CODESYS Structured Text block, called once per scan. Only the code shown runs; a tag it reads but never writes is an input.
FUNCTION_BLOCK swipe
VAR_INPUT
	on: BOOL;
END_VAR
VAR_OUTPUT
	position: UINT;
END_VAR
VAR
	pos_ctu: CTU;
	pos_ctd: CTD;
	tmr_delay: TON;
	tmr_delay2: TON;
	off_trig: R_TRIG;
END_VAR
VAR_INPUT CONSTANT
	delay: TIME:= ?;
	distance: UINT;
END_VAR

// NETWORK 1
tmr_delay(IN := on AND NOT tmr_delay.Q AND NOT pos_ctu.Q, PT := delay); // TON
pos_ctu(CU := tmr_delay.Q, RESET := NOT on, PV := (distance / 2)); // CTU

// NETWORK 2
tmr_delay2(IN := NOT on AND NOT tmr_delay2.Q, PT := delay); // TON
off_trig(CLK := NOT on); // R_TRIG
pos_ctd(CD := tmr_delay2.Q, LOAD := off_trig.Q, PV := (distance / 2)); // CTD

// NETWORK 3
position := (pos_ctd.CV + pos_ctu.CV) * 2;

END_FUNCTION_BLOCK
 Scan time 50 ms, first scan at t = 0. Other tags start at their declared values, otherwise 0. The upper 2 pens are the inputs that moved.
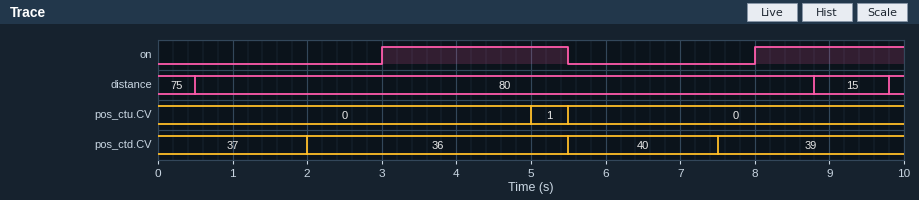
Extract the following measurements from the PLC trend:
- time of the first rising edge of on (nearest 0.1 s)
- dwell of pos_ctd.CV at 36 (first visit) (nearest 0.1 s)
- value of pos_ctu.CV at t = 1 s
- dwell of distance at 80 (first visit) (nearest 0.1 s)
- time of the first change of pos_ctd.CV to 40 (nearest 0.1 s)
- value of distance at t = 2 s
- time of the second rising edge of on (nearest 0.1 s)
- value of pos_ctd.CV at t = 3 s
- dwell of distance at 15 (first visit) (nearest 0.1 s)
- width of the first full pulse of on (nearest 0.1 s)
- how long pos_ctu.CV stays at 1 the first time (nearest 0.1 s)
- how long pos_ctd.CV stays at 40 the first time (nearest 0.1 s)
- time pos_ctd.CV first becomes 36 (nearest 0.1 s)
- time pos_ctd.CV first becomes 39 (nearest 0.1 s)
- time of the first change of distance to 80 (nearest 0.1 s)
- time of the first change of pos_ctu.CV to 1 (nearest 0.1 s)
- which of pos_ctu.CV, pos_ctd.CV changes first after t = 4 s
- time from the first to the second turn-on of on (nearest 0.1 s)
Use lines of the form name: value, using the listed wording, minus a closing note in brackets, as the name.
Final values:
time of the first rising edge of on: 3.0 s
dwell of pos_ctd.CV at 36 (first visit): 3.5 s
value of pos_ctu.CV at t = 1 s: 0
dwell of distance at 80 (first visit): 8.3 s
time of the first change of pos_ctd.CV to 40: 5.5 s
value of distance at t = 2 s: 80
time of the second rising edge of on: 8.0 s
value of pos_ctd.CV at t = 3 s: 36
dwell of distance at 15 (first visit): 1.0 s
width of the first full pulse of on: 2.5 s
how long pos_ctu.CV stays at 1 the first time: 0.5 s
how long pos_ctd.CV stays at 40 the first time: 2.0 s
time pos_ctd.CV first becomes 36: 2.0 s
time pos_ctd.CV first becomes 39: 7.5 s
time of the first change of distance to 80: 0.5 s
time of the first change of pos_ctu.CV to 1: 5.0 s
which of pos_ctu.CV, pos_ctd.CV changes first after t = 4 s: pos_ctu.CV
time from the first to the second turn-on of on: 5.0 s
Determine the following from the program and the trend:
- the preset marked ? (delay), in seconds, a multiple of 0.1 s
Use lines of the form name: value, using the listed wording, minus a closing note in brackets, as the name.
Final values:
the preset marked ? (delay), in seconds, a multiple of 0.1 s: 2.0 s
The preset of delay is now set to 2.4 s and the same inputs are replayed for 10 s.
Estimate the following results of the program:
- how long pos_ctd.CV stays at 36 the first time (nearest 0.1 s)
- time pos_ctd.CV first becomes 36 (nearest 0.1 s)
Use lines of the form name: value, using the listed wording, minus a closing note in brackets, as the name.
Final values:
how long pos_ctd.CV stays at 36 the first time: 3.1 s
time pos_ctd.CV first becomes 36: 2.4 s
